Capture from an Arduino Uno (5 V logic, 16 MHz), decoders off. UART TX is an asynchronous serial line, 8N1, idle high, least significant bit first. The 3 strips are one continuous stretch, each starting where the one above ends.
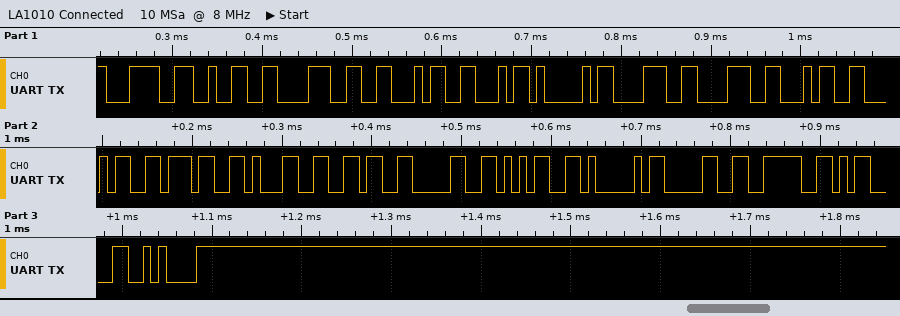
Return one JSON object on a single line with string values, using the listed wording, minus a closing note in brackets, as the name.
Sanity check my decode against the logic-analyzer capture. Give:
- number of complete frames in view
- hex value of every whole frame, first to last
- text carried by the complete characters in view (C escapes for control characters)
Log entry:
{"number of complete frames in view": "20", "hex value of every whole frame, first to last": "0x3C 0x32 0x38 0x46 0x46 0x41 0x38 0x38 0x34 0x34 0x37 0x31 0x36 0x30 0x35 0x41 0x30 0x3E 0x0D 0x0A", "text carried by the complete characters in view": "\"<28FFA884471605A0>\\r\\n\""}
